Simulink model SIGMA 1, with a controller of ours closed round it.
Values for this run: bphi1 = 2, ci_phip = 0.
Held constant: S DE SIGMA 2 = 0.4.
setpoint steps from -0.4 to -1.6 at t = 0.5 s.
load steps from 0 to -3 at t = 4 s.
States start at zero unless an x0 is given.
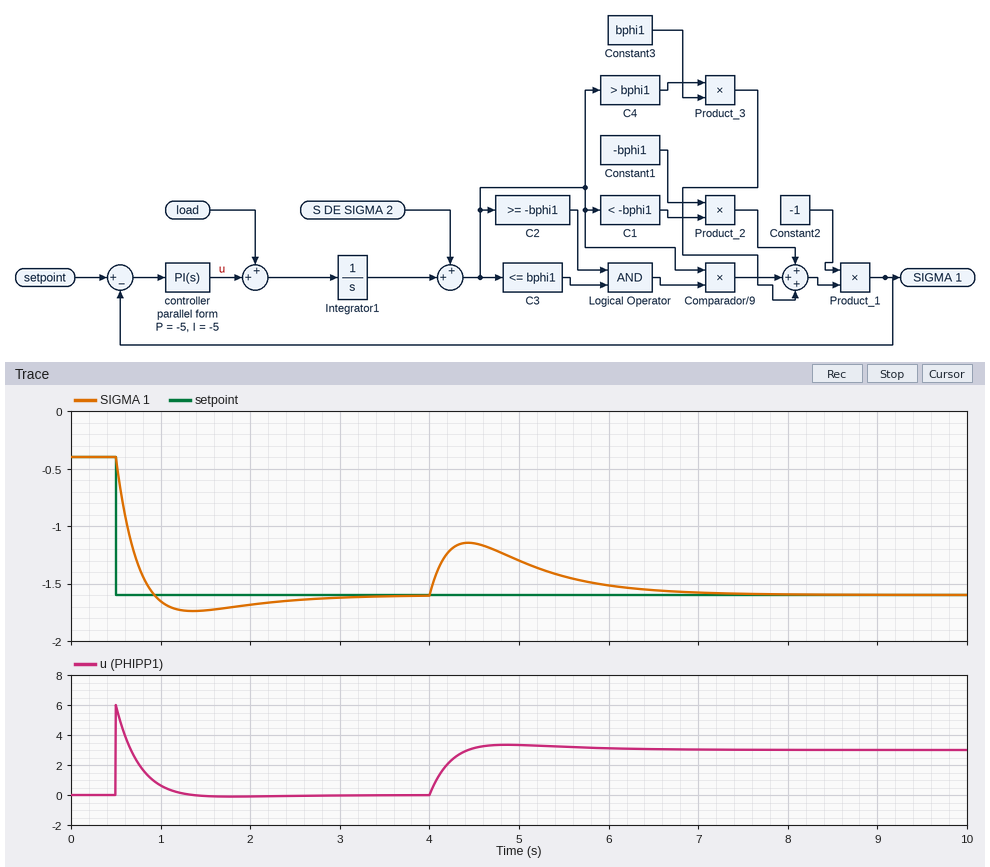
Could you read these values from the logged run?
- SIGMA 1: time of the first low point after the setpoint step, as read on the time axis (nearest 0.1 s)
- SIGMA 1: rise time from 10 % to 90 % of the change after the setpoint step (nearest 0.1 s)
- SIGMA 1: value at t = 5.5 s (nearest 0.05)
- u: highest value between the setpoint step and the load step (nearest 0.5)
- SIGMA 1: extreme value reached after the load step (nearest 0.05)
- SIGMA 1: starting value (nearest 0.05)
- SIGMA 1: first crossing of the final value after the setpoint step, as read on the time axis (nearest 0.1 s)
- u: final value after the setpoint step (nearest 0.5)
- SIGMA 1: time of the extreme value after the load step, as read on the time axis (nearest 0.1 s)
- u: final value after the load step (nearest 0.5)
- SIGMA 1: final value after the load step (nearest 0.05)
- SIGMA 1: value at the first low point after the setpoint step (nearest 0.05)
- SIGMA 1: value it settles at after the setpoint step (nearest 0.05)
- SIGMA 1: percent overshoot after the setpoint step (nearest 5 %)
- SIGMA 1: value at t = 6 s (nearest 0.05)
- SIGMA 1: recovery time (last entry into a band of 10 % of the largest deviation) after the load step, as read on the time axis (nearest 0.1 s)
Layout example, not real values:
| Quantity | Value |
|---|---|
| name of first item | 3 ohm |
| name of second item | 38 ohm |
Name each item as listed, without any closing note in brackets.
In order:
| Quantity | Value |
|---|---|
| SIGMA 1: time of the first low point after the setpoint step, as read on the time axis | 1.4 s |
| SIGMA 1: rise time from 10 % to 90 % of the change after the setpoint step | 0.3 s |
| SIGMA 1: value at t = 5.5 s | -1.45 |
| u: highest value between the setpoint step and the load step | 6.0 |
| SIGMA 1: extreme value reached after the load step | -1.15 |
| SIGMA 1: starting value | -0.40 |
| SIGMA 1: first crossing of the final value after the setpoint step, as read on the time axis | 0.9 s |
| u: final value after the setpoint step | 0.0 |
| SIGMA 1: time of the extreme value after the load step, as read on the time axis | 4.4 s |
| u: final value after the load step | 3.0 |
| SIGMA 1: final value after the load step | -1.60 |
| SIGMA 1: value at the first low point after the setpoint step | -1.75 |
| SIGMA 1: value it settles at after the setpoint step | -1.60 |
| SIGMA 1: percent overshoot after the setpoint step | 10 % |
| SIGMA 1: value at t = 6 s | -1.50 |
| SIGMA 1: recovery time (last entry into a band of 10 % of the largest deviation) after the load step, as read on the time axis | 6.4 s |
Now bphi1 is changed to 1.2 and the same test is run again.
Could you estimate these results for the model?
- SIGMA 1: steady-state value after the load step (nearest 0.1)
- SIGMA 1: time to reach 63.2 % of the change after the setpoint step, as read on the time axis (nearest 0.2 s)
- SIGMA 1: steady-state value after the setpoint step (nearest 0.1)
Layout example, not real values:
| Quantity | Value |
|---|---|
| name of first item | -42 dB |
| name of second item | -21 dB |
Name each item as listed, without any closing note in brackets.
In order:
| Quantity | Value |
|---|---|
| SIGMA 1: steady-state value after the load step | -1.2 |
| SIGMA 1: time to reach 63.2 % of the change after the setpoint step, as read on the time axis | 0.6 s |
| SIGMA 1: steady-state value after the setpoint step | -1.2 |
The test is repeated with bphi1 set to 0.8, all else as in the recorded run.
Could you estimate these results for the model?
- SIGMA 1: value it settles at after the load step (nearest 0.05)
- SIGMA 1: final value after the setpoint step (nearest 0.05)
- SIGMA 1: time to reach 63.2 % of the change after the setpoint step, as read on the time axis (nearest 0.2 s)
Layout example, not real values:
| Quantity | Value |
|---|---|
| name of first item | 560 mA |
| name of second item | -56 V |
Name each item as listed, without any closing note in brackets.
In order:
| Quantity | Value |
|---|---|
| SIGMA 1: value it settles at after the load step | -0.80 |
| SIGMA 1: final value after the setpoint step | -0.80 |
| SIGMA 1: time to reach 63.2 % of the change after the setpoint step, as read on the time axis | 0.6 s |
